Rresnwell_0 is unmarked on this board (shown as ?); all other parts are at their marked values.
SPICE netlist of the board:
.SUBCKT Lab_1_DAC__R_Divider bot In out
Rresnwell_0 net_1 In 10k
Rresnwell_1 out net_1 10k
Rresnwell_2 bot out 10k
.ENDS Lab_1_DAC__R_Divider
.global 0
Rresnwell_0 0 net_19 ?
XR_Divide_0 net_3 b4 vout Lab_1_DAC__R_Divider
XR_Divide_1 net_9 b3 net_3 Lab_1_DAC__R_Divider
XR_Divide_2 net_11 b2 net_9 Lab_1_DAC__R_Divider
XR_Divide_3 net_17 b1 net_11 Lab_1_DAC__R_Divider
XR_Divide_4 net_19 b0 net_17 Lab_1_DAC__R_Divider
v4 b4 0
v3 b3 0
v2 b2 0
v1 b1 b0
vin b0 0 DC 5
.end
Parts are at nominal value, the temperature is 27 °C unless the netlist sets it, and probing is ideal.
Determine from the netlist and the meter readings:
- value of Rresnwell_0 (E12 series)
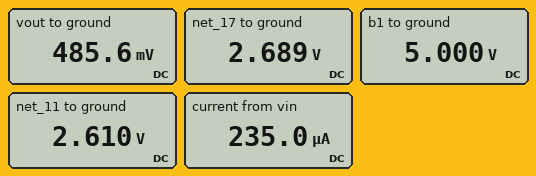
15 kΩ
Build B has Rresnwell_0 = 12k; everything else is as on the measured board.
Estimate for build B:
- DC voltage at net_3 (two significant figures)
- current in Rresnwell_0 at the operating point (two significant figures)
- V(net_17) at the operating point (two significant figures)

710 mV
120 µA
2.6 V
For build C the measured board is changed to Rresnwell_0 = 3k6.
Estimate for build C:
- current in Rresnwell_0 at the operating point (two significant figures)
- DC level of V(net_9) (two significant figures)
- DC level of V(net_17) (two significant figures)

160 µA
1.2 V
2.2 V
